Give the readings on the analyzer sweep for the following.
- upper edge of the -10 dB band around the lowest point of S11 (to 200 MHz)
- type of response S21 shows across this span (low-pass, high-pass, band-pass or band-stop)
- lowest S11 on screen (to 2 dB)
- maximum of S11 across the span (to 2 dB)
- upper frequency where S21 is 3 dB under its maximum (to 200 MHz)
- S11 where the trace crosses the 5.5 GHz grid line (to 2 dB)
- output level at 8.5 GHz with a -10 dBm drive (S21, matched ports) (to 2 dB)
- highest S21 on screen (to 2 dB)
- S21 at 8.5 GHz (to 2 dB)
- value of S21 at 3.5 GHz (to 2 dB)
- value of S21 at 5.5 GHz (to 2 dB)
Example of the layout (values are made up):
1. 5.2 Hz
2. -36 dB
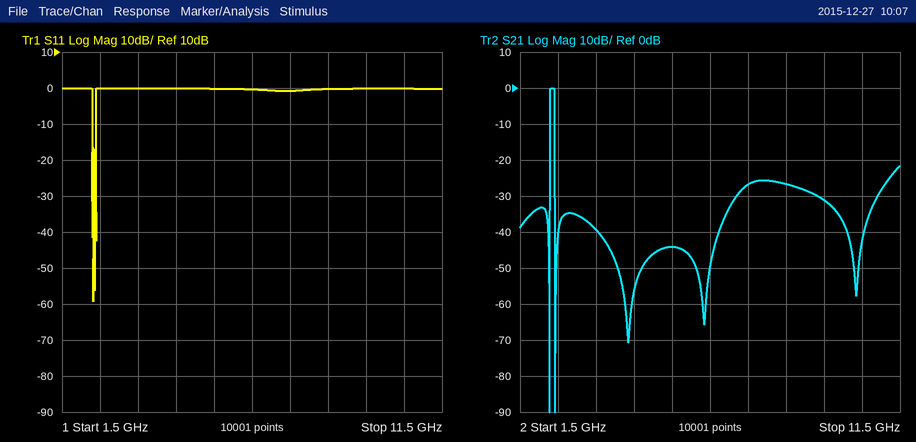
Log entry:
1. 2.4 GHz
2. band-pass
3. -60 dB
4. 0 dB
5. 2.4 GHz
6. 0 dB
7. -36 dBm
8. 0 dB
9. -26 dB
10. -40 dB
11. -44 dB
